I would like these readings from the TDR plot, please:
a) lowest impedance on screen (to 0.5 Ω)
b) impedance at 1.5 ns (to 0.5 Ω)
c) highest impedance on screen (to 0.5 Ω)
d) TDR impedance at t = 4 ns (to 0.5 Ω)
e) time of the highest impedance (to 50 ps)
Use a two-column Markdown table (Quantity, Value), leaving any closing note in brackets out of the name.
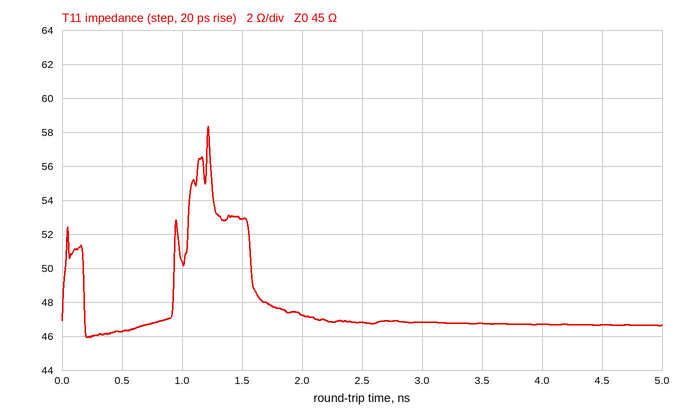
| Quantity | Value |
|---|---|
| lowest impedance on screen | 46.0 Ω |
| impedance at 1.5 ns | 53.0 Ω |
| highest impedance on screen | 58.5 Ω |
| TDR impedance at t = 4 ns | 46.5 Ω |
| time of the highest impedance | 1.20 ns |
